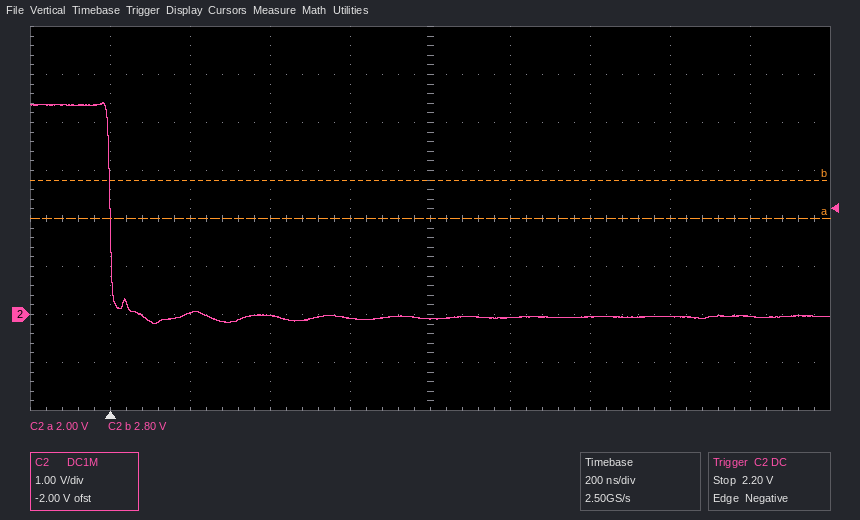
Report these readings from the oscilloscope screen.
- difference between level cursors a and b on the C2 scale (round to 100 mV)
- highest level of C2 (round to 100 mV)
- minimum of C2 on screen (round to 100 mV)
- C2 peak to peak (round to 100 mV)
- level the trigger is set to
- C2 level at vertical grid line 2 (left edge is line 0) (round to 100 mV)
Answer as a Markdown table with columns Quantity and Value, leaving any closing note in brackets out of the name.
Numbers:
| Quantity | Value |
|---|---|
| difference between level cursors a and b on the C2 scale | 800 mV |
| highest level of C2 | 4.4 V |
| minimum of C2 on screen | -200 mV |
| C2 peak to peak | 4.6 V |
| level the trigger is set to | 2.20 V |
| C2 level at vertical grid line 2 (left edge is line 0) | 0.0 V |
